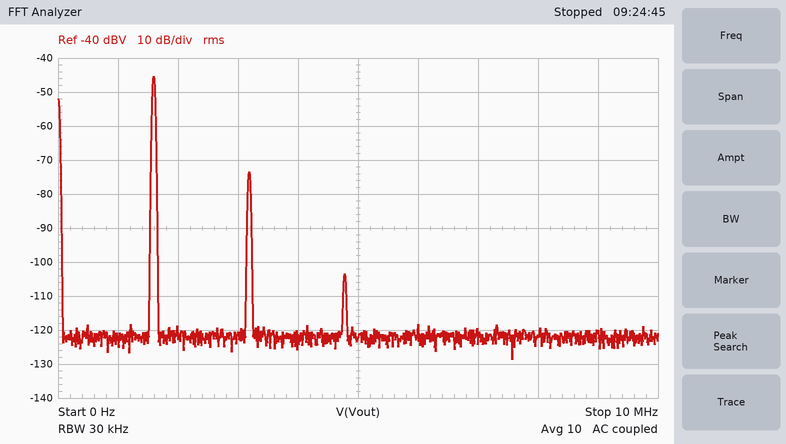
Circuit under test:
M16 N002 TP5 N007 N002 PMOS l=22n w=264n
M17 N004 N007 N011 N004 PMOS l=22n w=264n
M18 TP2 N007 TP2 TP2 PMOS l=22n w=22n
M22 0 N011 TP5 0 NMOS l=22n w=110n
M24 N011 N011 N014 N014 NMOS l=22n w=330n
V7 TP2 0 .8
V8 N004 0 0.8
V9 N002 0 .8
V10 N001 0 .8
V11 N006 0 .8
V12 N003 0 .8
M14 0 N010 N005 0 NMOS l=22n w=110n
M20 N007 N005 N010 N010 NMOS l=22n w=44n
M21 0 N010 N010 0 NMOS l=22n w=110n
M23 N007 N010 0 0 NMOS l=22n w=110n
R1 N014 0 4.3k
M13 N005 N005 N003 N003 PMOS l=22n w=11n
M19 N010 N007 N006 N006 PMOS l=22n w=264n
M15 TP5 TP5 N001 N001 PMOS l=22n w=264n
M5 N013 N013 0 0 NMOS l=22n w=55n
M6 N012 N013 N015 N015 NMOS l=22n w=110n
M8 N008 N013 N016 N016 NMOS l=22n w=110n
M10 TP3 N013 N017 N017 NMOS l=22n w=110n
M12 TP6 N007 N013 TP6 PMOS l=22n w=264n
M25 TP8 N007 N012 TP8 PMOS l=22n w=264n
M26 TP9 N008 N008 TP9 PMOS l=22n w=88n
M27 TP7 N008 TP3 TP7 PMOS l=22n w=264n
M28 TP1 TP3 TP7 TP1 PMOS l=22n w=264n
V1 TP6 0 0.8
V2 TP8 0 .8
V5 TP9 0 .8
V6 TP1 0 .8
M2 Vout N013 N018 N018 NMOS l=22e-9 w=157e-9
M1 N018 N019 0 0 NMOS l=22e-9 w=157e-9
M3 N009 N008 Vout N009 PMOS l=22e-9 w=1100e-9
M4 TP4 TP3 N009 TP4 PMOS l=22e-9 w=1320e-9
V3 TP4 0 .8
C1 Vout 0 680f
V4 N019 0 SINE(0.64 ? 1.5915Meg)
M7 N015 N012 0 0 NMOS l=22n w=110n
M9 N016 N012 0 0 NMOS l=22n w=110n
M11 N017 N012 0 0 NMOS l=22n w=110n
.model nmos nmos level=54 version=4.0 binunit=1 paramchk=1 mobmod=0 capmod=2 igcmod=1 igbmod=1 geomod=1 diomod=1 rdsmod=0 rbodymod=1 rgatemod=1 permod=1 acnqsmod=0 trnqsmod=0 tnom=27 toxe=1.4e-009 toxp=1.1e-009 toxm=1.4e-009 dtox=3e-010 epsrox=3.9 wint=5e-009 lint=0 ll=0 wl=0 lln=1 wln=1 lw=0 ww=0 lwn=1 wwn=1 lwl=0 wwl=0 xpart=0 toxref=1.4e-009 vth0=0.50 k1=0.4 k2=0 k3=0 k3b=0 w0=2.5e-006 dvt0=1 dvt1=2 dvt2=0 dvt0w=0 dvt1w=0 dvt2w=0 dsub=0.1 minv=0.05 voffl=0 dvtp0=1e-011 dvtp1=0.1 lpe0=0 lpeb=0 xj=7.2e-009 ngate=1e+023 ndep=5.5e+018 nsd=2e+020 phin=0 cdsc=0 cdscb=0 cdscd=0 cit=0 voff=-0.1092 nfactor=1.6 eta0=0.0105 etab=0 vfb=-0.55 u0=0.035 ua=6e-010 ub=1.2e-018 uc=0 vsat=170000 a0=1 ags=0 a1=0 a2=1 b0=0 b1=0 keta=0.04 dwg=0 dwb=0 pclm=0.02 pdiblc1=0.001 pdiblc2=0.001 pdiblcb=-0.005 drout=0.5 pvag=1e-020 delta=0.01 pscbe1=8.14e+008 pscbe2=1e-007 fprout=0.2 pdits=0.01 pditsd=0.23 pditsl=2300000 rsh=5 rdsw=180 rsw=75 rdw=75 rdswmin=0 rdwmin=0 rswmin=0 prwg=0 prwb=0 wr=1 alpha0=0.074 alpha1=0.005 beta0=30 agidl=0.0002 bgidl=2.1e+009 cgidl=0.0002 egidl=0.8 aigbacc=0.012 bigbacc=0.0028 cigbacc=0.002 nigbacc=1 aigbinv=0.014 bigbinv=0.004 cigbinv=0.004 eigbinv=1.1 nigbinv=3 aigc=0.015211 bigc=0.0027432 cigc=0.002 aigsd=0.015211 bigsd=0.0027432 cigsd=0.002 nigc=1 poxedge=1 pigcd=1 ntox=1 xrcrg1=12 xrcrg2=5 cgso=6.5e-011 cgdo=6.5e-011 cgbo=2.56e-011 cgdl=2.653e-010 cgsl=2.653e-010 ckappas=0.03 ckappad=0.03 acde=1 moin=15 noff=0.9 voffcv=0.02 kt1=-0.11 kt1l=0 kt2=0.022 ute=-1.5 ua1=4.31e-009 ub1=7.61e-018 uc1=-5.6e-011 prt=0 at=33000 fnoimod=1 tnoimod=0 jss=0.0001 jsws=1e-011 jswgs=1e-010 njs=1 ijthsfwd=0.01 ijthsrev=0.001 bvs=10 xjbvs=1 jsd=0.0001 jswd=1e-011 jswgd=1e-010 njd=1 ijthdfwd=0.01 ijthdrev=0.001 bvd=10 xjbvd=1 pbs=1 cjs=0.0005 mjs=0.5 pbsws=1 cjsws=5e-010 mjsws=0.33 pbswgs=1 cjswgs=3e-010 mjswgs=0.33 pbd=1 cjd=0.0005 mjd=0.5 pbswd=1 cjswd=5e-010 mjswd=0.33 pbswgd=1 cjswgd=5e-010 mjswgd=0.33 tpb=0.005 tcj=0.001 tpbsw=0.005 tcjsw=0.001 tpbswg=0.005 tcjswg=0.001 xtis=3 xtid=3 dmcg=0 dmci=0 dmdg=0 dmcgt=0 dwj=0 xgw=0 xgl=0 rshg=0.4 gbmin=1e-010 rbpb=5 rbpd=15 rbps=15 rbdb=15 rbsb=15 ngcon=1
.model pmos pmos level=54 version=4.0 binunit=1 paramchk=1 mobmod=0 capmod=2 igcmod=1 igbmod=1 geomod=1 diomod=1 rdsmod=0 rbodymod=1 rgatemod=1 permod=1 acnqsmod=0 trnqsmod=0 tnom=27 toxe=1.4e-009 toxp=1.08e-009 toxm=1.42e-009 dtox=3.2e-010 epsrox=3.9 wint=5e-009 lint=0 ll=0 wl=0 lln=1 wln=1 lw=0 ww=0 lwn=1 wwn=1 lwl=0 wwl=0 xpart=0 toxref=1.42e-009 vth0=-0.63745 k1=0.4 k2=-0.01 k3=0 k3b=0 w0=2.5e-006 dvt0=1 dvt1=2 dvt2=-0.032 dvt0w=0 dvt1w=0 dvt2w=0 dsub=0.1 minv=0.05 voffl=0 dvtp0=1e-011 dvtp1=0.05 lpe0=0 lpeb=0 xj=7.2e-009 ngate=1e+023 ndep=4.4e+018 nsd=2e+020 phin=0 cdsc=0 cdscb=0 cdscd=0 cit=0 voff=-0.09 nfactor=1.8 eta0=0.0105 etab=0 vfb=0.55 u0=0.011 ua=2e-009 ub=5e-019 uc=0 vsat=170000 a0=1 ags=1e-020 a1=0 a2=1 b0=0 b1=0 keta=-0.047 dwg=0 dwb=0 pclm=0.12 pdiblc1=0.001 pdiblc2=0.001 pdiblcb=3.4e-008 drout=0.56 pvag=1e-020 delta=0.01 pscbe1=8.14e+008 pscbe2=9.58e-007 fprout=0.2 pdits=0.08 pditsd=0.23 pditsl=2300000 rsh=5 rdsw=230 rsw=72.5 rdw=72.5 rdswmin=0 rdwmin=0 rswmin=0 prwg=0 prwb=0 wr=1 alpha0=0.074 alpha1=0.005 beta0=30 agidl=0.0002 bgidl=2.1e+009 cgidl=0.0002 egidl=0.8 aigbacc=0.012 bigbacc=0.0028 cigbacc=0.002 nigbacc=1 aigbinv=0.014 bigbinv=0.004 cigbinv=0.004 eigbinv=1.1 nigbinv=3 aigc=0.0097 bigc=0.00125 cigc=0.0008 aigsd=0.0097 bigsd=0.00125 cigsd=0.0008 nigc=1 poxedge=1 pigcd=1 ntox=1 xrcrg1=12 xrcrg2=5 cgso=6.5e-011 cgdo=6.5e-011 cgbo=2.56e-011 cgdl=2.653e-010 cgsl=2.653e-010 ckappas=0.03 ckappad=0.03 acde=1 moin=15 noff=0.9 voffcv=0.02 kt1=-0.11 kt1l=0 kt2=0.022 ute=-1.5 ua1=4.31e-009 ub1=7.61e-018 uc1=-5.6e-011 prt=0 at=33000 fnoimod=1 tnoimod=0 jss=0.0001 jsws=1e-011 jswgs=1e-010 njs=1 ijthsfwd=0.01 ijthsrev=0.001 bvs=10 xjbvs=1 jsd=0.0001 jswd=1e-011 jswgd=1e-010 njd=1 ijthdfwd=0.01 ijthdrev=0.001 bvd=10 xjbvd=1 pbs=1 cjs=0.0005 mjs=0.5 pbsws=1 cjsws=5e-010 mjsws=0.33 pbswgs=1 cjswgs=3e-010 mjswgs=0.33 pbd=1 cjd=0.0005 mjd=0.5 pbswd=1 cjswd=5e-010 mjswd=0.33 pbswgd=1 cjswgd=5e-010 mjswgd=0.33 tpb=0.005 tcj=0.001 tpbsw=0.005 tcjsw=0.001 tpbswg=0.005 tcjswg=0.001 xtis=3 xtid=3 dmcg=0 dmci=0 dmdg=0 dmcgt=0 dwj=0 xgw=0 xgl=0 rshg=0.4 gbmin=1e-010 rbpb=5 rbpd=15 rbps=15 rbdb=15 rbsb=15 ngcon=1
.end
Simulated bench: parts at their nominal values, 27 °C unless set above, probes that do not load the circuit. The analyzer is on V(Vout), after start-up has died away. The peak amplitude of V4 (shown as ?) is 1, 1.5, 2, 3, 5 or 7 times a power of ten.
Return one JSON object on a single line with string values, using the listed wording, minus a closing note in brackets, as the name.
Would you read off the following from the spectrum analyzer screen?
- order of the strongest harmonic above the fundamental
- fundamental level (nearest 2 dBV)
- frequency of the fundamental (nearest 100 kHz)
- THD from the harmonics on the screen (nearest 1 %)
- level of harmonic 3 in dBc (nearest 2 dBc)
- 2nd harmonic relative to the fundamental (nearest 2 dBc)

{"order of the strongest harmonic above the fundamental": "2", "fundamental level": "-46 dBV", "frequency of the fundamental": "1.6 MHz", "THD from the harmonics on the screen": "4 %", "level of harmonic 3 in dBc": "-58 dBc", "2nd harmonic relative to the fundamental": "-28 dBc"}
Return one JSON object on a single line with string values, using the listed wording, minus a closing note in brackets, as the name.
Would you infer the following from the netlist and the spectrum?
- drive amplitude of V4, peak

{"drive amplitude of V4, peak": "15 mV"}
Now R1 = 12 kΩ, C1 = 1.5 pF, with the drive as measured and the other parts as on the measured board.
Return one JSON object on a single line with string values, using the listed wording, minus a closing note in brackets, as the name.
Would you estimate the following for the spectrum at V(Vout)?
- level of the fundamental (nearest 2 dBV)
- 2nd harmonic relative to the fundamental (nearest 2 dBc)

{"level of the fundamental": "-54 dBV", "2nd harmonic relative to the fundamental": "-32 dBc"}
